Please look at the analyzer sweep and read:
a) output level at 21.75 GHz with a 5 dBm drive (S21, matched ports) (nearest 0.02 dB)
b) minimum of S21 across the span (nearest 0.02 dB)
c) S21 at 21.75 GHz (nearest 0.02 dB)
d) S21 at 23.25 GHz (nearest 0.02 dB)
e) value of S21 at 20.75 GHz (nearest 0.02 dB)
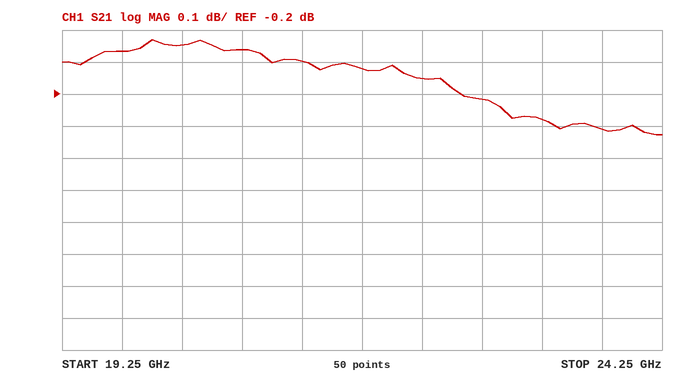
4.88 dBm
-0.32 dB
-0.12 dB
-0.28 dB
-0.06 dB
